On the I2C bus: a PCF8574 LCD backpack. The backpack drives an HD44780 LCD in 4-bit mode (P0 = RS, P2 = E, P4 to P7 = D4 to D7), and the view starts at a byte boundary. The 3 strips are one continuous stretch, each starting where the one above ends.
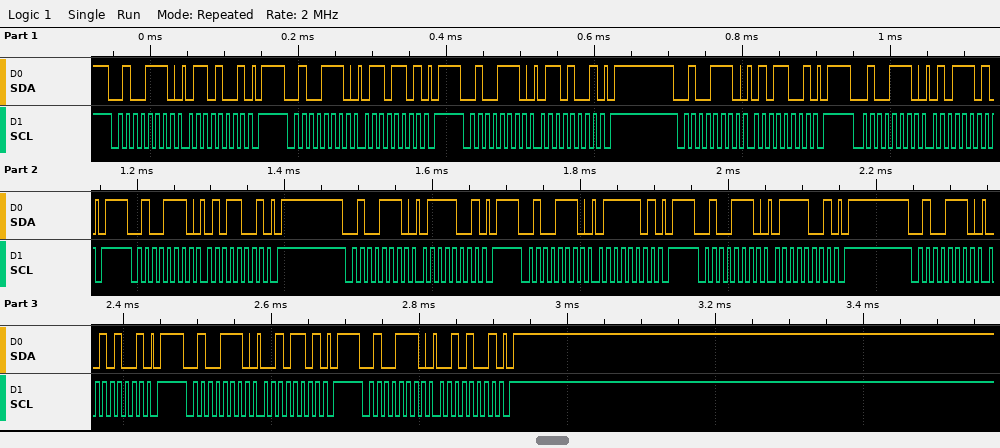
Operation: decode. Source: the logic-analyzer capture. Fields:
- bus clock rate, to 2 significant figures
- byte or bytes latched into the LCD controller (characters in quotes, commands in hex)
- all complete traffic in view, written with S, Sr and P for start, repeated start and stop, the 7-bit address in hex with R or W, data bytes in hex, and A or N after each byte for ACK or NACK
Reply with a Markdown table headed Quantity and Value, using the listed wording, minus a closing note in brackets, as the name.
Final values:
| Quantity | Value |
|---|---|
| bus clock rate, to 2 significant figures | 100 kHz |
| byte or bytes latched into the LCD controller | 'e' 'r' |
| all complete traffic in view, written with S, Sr and P for start, repeated start and stop, the 7-bit address in hex with R or W, data bytes in hex, and A or N after each byte for ACK or NACK | S 27W A 69 A P S 27W A 6D A P S 27W A 69 A P S 27W A 59 A P S 27W A 5D A P S 27W A 59 A P S 27W A 79 A P S 27W A 7D A P S 27W A 79 A P S 27W A 29 A P S 27W A 2D A P S 27W A 29 A P |
